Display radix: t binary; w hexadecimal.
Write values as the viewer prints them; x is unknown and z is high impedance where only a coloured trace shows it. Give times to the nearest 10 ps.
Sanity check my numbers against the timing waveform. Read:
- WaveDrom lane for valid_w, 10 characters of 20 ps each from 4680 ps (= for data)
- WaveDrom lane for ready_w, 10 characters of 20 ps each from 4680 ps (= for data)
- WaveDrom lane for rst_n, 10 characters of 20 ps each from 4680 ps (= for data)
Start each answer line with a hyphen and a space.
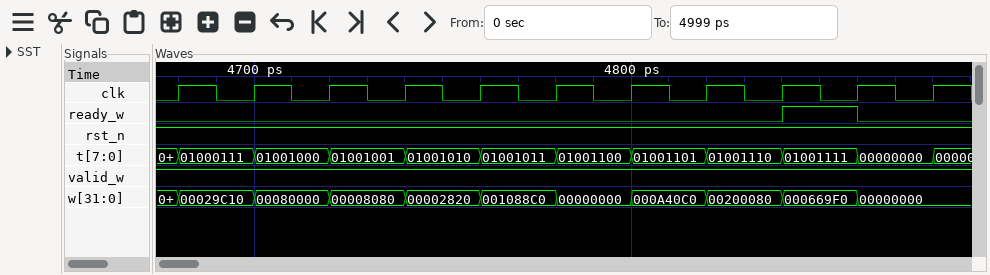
- {name: 'valid_w', wave: '1.........'}
- {name: 'ready_w', wave: '0.......10'}
- {name: 'rst_n', wave: '1.........'}
